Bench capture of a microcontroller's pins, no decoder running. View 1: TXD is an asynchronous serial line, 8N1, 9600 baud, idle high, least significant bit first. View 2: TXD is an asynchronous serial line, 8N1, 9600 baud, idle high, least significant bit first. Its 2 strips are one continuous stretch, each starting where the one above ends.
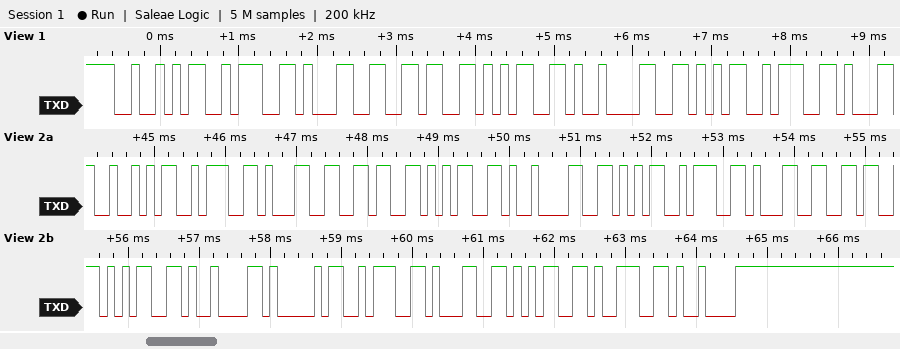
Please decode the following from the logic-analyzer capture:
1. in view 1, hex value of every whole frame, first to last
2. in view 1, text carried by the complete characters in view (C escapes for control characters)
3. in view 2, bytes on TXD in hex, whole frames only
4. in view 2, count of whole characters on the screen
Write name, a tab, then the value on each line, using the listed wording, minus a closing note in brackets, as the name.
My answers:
in view 1, hex value of every whole frame, first to last	0x52 0x3A 0x31 0x36 0x35 0x09 0x56 0x3A
in view 1, text carried by the complete characters in view	"R:165\tV:"
in view 2, bytes on TXD in hex, whole frames only	52 3A 31 36 35 09 56 3A 31 36 35 09 41 3A 31 35 39 09
in view 2, count of whole characters on the screen	18
